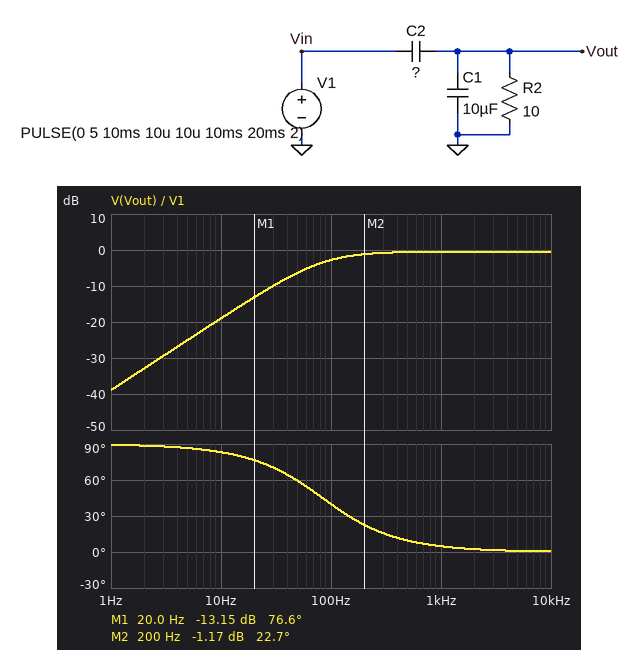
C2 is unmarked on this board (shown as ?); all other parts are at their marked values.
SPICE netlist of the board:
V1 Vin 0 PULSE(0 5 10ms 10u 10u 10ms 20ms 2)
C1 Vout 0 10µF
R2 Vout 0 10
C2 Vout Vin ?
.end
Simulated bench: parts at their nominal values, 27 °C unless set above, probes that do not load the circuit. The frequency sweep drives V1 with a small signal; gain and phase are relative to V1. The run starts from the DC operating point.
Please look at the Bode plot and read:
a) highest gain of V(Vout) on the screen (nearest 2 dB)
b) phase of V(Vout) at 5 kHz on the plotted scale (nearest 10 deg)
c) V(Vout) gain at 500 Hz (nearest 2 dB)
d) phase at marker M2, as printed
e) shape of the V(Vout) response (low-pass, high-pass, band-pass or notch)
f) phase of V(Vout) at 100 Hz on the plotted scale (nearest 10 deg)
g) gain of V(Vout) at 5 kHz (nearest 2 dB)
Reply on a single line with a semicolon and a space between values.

0 dB; 0 deg; 0 dB; 22.7 deg; high-pass; 40 deg; 0 dB
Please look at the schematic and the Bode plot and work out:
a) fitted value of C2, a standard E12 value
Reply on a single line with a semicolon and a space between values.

180 µF
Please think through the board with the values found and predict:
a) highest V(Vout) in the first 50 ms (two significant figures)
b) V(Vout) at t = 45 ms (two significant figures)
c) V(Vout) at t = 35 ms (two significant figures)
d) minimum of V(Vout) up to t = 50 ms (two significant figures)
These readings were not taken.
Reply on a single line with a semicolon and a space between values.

4.7 V; -340 mV; 340 mV; -4.7 V
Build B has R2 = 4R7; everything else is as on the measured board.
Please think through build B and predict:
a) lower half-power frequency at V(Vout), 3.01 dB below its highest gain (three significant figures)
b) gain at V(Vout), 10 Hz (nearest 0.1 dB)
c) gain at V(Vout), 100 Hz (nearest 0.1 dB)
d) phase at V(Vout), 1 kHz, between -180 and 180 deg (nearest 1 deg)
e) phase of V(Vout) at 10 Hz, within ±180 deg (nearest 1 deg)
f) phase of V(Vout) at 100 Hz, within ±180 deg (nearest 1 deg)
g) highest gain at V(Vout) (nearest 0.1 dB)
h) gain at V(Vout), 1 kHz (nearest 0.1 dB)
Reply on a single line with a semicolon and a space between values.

178 Hz; -25.5 dB; -6.7 dB; 10 deg; 87 deg; 61 deg; -0.5 dB; -0.6 dB
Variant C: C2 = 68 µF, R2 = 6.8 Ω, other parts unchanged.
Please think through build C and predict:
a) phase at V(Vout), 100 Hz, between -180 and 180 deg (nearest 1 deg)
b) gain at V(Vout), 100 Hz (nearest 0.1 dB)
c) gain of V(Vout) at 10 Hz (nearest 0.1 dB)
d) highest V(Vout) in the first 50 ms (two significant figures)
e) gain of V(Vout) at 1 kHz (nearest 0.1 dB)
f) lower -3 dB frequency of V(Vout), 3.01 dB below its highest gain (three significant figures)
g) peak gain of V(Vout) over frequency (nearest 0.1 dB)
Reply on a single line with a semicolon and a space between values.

72 deg; -11.2 dB; -30.7 dB; 4.3 V; -1.6 dB; 300 Hz; -1.2 dB
